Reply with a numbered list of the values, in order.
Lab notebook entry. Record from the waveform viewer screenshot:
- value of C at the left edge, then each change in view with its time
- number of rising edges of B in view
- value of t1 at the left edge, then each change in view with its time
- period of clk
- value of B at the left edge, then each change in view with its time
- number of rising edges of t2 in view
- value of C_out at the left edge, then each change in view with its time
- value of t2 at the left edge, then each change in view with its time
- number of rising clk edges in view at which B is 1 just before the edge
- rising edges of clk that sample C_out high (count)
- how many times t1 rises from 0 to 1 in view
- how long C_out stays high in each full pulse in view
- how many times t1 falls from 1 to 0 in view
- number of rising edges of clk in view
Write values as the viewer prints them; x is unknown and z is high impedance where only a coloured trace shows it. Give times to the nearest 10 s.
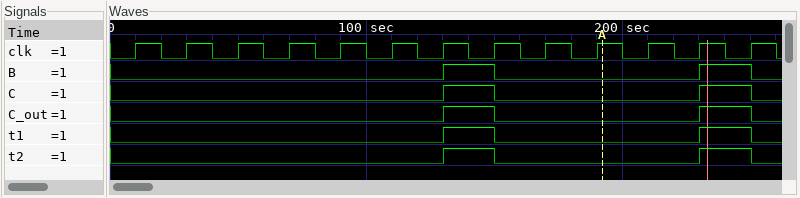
1. 0, 1 at 130 s, 0 at 150 s, 1 at 230 s, 0 at 250 s
2. 2
3. 0, 1 at 130 s, 0 at 150 s, 1 at 230 s, 0 at 250 s
4. 20 s
5. 0, 1 at 130 s, 0 at 150 s, 1 at 230 s, 0 at 250 s
6. 2
7. 0, 1 at 130 s, 0 at 150 s, 1 at 230 s, 0 at 250 s
8. 0, 1 at 130 s, 0 at 150 s, 1 at 230 s, 0 at 250 s
9. 2
10. 2
11. 2
12. 20 s, 20 s
13. 2
14. 13
